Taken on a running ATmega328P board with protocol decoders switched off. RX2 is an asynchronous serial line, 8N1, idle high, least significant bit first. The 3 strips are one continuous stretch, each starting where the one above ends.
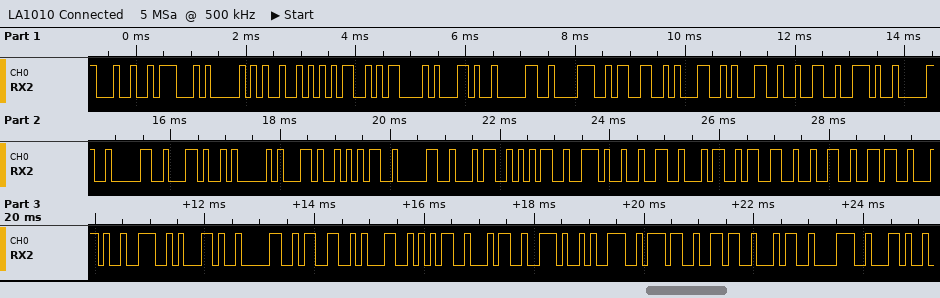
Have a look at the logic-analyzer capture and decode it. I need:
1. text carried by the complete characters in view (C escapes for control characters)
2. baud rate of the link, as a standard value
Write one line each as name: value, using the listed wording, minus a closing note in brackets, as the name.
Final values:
text carried by the complete characters in view: "$GPRMC,083112.00,A,5045.24326,N,03154.97648,"
baud rate of the link, as a standard value: 9600 baud
